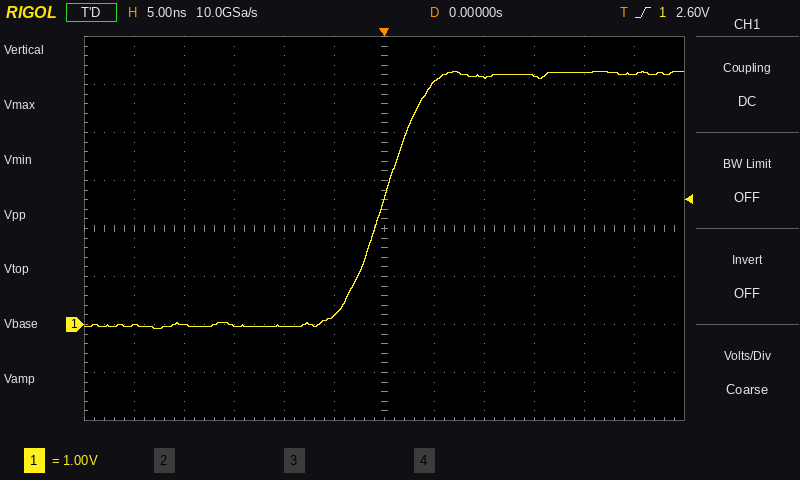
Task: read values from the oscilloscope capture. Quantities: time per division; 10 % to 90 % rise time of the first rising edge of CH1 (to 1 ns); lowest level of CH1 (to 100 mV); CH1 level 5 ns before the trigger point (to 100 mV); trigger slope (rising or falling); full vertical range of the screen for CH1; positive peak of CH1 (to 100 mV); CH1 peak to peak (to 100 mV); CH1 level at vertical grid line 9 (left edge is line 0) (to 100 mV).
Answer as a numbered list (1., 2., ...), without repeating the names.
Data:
1. 5 ns
2. 8 ns
3. -100 mV
4. 200 mV
5. rising
6. 8 V
7. 5.3 V
8. 5.4 V
9. 5.2 V
